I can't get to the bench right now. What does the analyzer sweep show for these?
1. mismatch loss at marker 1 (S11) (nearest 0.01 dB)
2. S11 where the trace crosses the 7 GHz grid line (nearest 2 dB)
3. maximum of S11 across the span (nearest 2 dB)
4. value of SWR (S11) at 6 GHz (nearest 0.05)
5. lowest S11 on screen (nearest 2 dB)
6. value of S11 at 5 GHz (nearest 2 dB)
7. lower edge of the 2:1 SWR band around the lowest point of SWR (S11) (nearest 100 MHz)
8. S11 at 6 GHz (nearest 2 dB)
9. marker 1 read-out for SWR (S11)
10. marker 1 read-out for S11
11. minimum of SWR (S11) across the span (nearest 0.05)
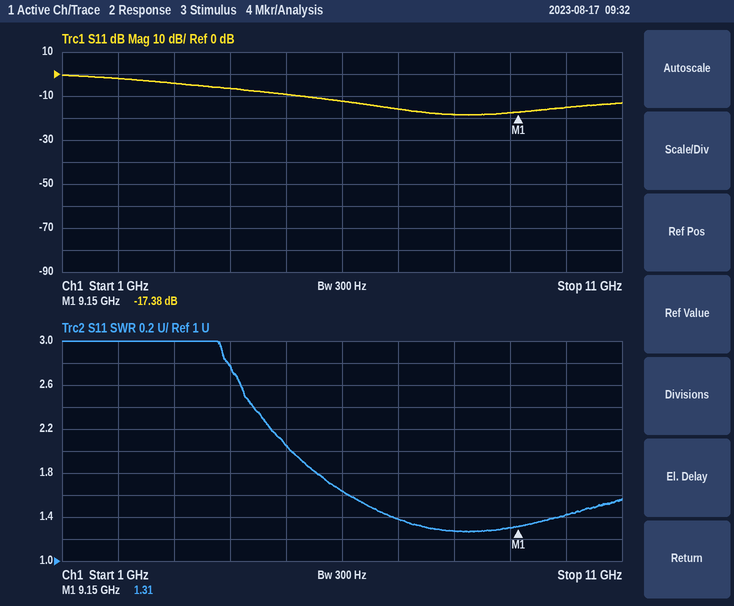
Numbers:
0.08 dB
-16 dB
0 dB
1.65
-18 dB
-10 dB
5.1 GHz
-12 dB
1.31
-17.38 dB
1.25
